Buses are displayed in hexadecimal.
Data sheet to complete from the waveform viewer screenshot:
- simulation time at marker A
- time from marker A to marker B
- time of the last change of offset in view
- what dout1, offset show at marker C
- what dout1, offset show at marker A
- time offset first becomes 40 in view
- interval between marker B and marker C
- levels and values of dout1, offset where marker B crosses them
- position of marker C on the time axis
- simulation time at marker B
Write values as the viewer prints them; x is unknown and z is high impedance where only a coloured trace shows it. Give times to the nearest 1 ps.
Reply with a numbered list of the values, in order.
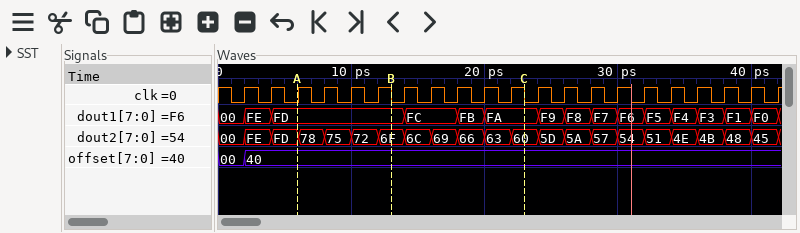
1. 6 ps
2. 7 ps
3. 2 ps
4. dout1=FA, offset=40
5. dout1=FD, offset=40
6. 2 ps
7. 10 ps
8. dout1=FD, offset=40
9. 23 ps
10. 13 ps
